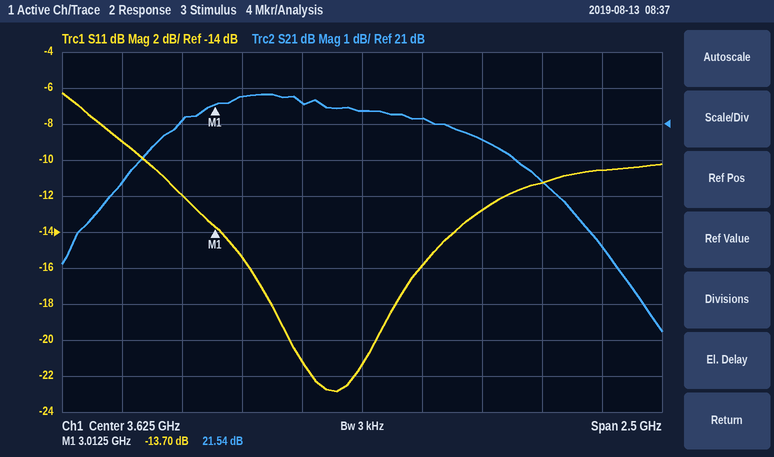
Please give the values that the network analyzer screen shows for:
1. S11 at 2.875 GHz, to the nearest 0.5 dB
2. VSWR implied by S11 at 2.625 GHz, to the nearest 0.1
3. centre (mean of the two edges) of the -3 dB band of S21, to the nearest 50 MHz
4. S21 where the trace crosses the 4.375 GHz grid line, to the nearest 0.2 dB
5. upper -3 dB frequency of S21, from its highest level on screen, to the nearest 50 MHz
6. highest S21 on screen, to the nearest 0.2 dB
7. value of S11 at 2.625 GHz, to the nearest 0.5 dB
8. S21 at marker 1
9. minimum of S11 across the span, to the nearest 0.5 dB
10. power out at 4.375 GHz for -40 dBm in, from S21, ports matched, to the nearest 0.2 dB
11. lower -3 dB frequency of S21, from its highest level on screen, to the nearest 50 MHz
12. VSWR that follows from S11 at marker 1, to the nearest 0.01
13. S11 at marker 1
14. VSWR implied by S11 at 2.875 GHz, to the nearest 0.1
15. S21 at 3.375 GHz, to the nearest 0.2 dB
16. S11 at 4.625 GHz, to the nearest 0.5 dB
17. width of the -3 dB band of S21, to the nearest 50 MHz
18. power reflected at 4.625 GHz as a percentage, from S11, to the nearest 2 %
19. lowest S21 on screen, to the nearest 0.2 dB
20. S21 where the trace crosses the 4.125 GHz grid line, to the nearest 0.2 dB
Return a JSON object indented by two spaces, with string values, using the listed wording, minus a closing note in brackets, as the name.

{
  "S11 at 2.875 GHz, to the nearest 0.5 dB": "-12.0 dB",
  "VSWR implied by S11 at 2.625 GHz, to the nearest 0.1": "2.1",
  "centre (mean of the two edges) of the -3 dB band of S21, to the nearest 50 MHz": "3.50 GHz",
  "S21 where the trace crosses the 4.375 GHz grid line, to the nearest 0.2 dB": "19.4 dB",
  "upper -3 dB frequency of S21, from its highest level on screen, to the nearest 50 MHz": "4.45 GHz",
  "highest S21 on screen, to the nearest 0.2 dB": "21.8 dB",
  "value of S11 at 2.625 GHz, to the nearest 0.5 dB": "-9.0 dB",
  "S21 at marker 1": "21.54 dB",
  "minimum of S11 across the span, to the nearest 0.5 dB": "-23.0 dB",
  "power out at 4.375 GHz for -40 dBm in, from S21, ports matched, to the nearest 0.2 dB": "-20.6 dBm",
  "lower -3 dB frequency of S21, from its highest level on screen, to the nearest 50 MHz": "2.55 GHz",
  "VSWR that follows from S11 at marker 1, to the nearest 0.01": "1.52",
  "S11 at marker 1": "-13.70 dB",
  "VSWR implied by S11 at 2.875 GHz, to the nearest 0.1": "1.7",
  "S21 at 3.375 GHz, to the nearest 0.2 dB": "21.6 dB",
  "S11 at 4.625 GHz, to the nearest 0.5 dB": "-10.5 dB",
  "width of the -3 dB band of S21, to the nearest 50 MHz": "1.90 GHz",
  "power reflected at 4.625 GHz as a percentage, from S11, to the nearest 2 %": "8 %",
  "lowest S21 on screen, to the nearest 0.2 dB": "15.2 dB",
  "S21 where the trace crosses the 4.125 GHz grid line, to the nearest 0.2 dB": "20.6 dB"
}
